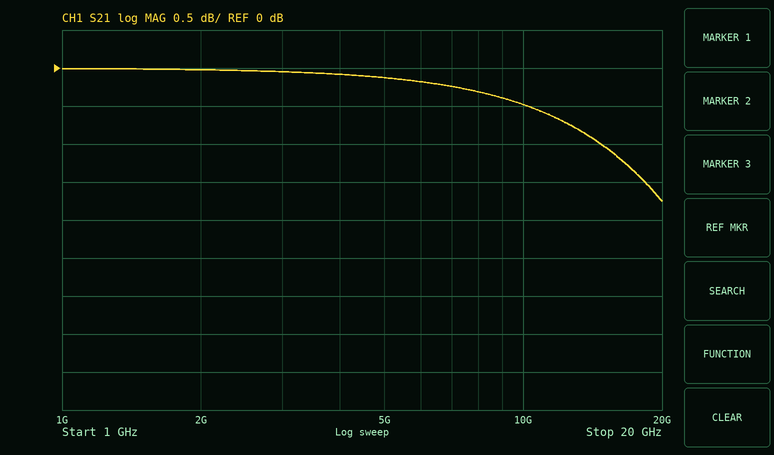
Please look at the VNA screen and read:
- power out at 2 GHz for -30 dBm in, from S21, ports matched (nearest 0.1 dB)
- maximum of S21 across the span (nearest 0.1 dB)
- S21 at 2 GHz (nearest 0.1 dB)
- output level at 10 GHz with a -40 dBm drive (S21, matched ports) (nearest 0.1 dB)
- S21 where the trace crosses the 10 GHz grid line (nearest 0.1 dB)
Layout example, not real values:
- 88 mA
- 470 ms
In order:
- -30.0 dBm
- 0.0 dB
- 0.0 dB
- -40.5 dBm
- -0.5 dB
